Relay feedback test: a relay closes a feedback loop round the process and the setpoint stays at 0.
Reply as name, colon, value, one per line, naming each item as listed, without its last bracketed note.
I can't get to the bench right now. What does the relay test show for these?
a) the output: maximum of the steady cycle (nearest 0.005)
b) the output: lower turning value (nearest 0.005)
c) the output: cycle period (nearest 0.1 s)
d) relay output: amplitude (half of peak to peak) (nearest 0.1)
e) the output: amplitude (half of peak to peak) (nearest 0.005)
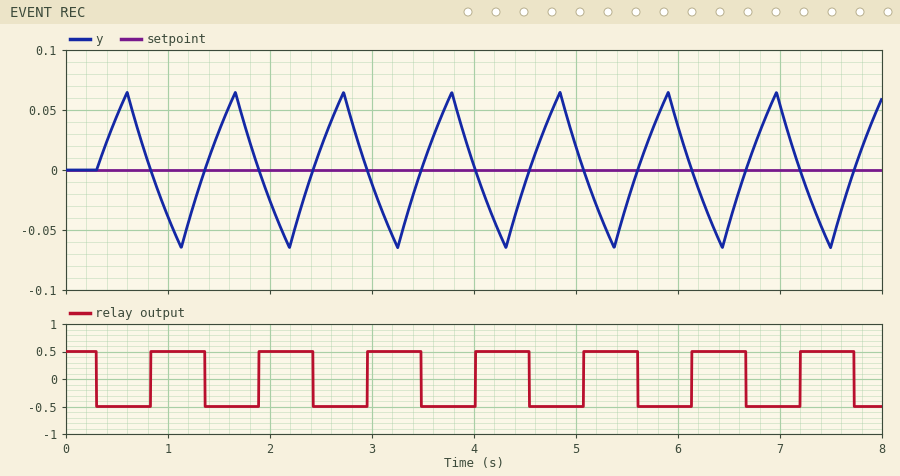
the output: maximum of the steady cycle: 0.065
the output: lower turning value: -0.065
the output: cycle period: 1.1 s
relay output: amplitude (half of peak to peak): 0.5
the output: amplitude (half of peak to peak): 0.065
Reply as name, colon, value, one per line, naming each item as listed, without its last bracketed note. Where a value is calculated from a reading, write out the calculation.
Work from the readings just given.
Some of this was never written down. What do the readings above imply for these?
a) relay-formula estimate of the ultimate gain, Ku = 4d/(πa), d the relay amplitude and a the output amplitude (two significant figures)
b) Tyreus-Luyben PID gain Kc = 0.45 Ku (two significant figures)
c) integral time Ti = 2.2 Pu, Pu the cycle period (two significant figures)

relay-formula estimate of the ultimate gain, Ku = 4d/(πa), d the relay amplitude and a the output amplitude: 4 × 0.5 / (π × 0.065) = 9.8
Tyreus-Luyben PID gain Kc = 0.45 Ku: 0.45 × 9.8 = 4.4
integral time Ti = 2.2 Pu, Pu the cycle period: 2.2 × 1.1 = 2.4 s
